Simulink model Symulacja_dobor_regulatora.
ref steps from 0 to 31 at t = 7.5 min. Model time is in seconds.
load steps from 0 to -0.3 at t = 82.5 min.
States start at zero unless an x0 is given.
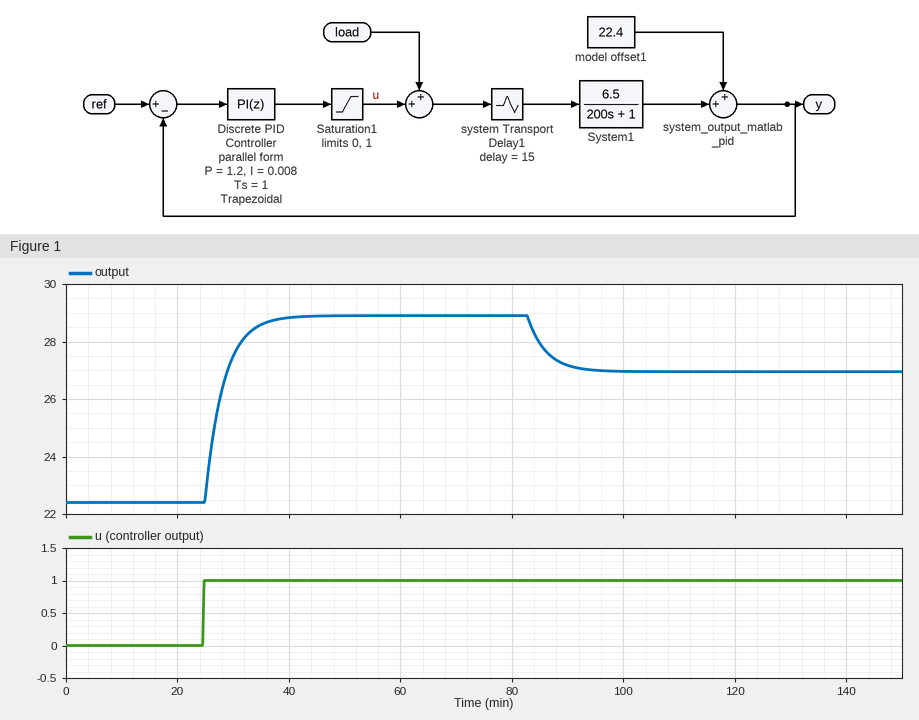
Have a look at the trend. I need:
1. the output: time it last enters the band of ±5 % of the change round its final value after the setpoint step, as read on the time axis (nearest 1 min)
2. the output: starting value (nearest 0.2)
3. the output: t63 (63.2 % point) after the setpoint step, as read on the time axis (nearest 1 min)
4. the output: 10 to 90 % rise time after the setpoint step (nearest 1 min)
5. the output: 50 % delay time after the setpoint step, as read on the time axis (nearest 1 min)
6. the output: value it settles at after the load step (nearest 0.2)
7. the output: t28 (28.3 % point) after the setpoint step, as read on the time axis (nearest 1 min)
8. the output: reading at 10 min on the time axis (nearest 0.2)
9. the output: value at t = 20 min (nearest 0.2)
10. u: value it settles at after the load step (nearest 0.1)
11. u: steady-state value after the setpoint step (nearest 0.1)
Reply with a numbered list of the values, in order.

1. 35 min
2. 22.4
3. 28 min
4. 7 min
5. 27 min
6. 27.0
7. 26 min
8. 22.4
9. 22.4
10. 1.0
11. 1.0
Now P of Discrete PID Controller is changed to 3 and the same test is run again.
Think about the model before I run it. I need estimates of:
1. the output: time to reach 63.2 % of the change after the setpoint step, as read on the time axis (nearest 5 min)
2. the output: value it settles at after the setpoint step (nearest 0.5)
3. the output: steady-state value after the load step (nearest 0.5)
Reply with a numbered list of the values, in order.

1. 25 min
2. 29.0
3. 27.0
